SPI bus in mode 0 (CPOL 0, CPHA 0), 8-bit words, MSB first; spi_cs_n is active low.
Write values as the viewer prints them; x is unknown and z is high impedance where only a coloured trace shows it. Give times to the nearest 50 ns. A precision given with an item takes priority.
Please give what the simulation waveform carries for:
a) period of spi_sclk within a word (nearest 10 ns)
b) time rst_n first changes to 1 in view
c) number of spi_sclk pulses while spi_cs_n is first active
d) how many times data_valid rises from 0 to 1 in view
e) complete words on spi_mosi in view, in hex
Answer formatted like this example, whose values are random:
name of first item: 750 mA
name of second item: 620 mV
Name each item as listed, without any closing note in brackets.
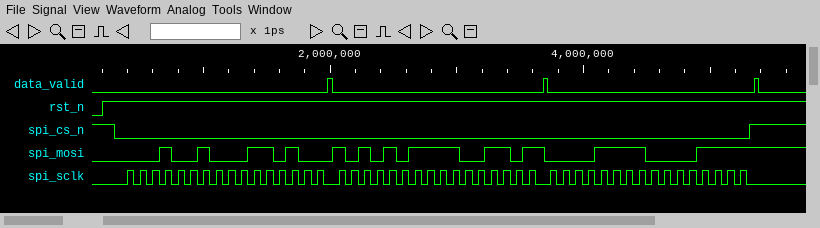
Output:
period of spi_sclk within a word: 100 ns
time rst_n first changes to 1 in view: 200 ns
number of spi_sclk pulses while spi_cs_n is first active: 48
how many times data_valid rises from 0 to 1 in view: 3
complete words on spi_mosi in view, in hex: 12, 34, AB, CD, 0F, 0F
